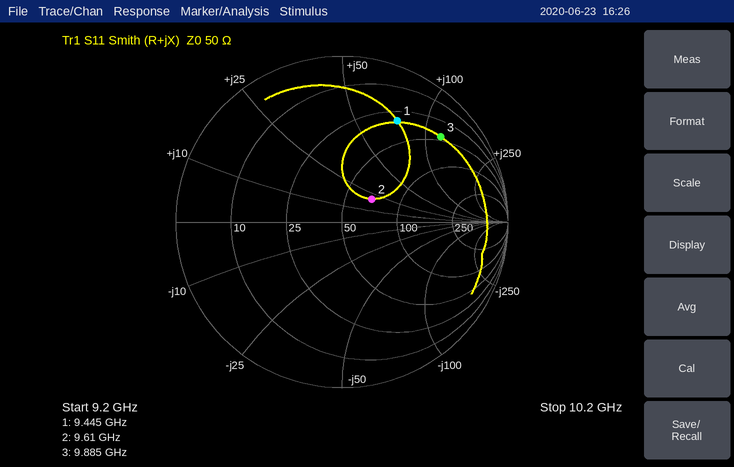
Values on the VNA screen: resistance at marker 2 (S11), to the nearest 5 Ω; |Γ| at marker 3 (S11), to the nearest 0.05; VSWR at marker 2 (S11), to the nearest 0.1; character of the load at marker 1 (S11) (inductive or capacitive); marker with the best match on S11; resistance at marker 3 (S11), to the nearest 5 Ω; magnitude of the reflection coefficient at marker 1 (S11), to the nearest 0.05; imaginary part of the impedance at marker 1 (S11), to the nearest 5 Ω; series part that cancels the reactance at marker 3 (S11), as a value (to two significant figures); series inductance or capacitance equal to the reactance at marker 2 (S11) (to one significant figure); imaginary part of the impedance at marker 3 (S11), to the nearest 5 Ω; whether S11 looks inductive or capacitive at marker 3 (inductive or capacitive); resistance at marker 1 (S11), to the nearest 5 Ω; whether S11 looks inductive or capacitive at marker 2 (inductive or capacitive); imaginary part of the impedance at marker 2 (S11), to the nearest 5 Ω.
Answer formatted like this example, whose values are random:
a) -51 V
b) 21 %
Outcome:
a) 70 Ω
b) 0.80
c) 1.6
d) inductive
e) marker 2
f) 45 Ω
g) 0.70
h) +75 Ω
i) 130 fF
j) 300 pH
k) +120 Ω
l) inductive
m) 30 Ω
n) inductive
o) +20 Ω
